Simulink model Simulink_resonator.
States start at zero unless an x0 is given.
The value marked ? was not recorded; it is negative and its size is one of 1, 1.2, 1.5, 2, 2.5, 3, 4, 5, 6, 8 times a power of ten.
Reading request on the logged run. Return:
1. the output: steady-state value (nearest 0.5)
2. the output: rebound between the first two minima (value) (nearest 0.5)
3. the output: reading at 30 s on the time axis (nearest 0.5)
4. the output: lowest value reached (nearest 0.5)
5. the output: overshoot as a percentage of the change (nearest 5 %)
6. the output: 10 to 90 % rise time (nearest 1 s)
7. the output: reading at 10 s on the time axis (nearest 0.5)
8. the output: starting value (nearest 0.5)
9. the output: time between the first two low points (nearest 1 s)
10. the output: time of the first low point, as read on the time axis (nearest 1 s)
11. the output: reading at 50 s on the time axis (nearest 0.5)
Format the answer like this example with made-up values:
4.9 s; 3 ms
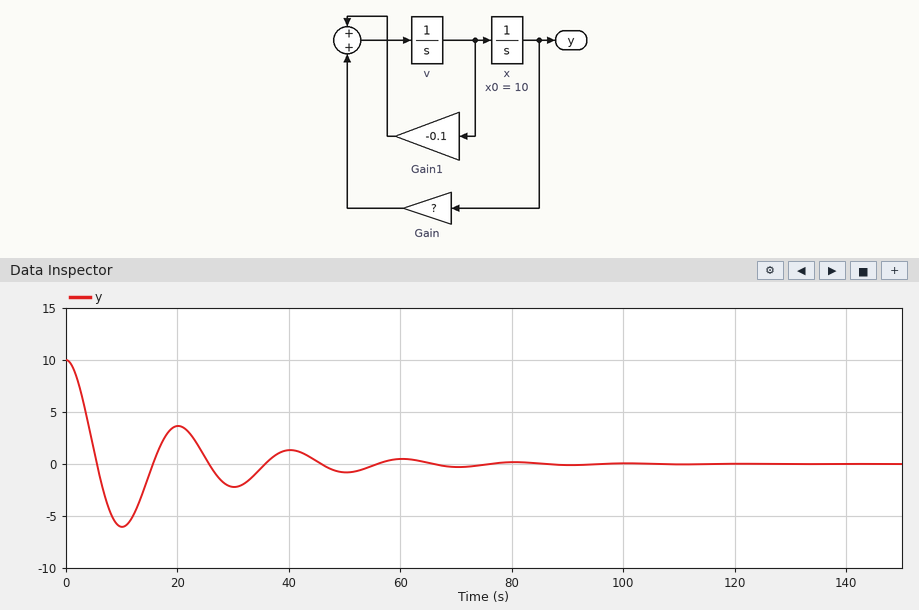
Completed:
0.0; 3.5; -2.0; -6.0; 60 %; 4 s; -6.0; 10.0; 20 s; 10 s; -1.0
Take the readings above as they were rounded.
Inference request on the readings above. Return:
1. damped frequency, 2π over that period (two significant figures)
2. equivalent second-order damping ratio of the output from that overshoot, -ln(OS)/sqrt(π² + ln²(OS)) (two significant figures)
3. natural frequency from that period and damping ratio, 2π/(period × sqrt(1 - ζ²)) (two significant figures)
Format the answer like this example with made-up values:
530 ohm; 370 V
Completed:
0.31 rad/s; 0.16; 0.32 rad/s
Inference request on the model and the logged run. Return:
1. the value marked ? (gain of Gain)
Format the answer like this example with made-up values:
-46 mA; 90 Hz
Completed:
-0.1
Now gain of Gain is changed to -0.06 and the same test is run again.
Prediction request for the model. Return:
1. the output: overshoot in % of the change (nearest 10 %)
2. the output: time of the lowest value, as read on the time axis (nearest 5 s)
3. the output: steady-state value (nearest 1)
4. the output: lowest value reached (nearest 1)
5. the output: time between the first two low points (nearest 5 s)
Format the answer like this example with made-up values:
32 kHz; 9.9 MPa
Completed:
50 %; 15 s; 0; -5; 25 s
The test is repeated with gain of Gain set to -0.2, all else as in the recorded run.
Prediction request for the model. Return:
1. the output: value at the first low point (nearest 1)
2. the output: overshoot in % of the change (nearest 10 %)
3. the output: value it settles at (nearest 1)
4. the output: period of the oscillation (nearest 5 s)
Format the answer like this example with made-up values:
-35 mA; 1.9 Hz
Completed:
-7; 70 %; 0; 15 s
